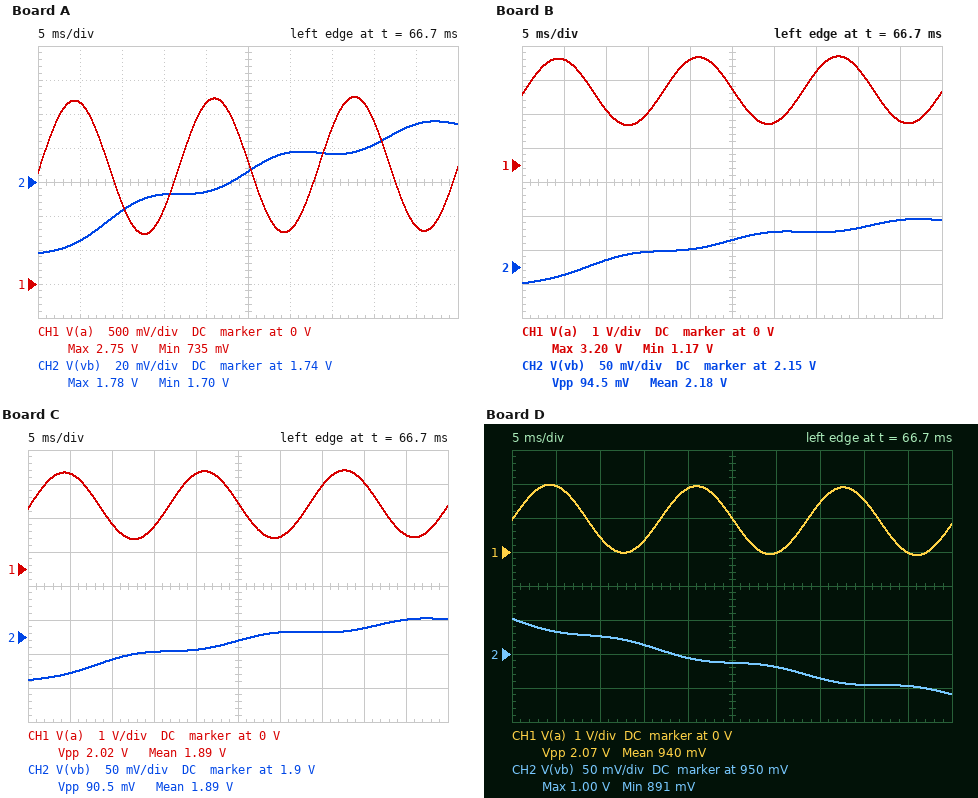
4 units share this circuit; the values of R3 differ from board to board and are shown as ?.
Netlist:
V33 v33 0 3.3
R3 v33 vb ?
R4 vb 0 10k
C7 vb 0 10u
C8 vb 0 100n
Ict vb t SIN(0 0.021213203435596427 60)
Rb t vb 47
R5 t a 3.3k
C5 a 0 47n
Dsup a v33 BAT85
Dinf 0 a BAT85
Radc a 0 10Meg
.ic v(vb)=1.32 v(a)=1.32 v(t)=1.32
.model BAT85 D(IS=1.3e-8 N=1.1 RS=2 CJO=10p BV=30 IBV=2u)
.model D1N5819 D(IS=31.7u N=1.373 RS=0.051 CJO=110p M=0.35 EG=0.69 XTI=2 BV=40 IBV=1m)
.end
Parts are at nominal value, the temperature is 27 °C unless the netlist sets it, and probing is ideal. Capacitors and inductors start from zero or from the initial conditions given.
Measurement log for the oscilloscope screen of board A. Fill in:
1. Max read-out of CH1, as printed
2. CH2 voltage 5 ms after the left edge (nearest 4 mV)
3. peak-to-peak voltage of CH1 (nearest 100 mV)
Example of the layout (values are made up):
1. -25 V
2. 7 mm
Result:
1. 2.75 V
2. 1.704 V
3. 2.0 V
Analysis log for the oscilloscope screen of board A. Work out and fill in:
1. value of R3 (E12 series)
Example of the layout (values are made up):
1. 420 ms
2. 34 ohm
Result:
1. 8.2 kΩ
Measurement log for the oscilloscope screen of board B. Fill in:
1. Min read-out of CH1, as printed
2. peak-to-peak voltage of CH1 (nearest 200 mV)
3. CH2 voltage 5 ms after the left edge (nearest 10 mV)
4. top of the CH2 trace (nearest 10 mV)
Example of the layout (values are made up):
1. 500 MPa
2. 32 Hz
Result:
1. 1.17 V
2. 2.0 V
3. 2.14 V
4. 2.22 V
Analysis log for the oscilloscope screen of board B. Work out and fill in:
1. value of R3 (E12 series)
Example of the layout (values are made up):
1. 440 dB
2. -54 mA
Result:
1. 4.7 kΩ
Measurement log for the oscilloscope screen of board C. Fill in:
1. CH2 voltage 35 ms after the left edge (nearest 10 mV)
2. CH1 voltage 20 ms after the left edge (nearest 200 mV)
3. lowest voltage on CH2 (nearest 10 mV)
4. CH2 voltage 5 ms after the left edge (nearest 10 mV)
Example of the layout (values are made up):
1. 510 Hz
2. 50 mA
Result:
1. 1.91 V
2. 2.8 V
3. 1.84 V
4. 1.85 V
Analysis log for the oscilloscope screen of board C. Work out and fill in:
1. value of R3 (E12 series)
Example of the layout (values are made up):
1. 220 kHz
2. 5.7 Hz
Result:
1. 6.8 kΩ
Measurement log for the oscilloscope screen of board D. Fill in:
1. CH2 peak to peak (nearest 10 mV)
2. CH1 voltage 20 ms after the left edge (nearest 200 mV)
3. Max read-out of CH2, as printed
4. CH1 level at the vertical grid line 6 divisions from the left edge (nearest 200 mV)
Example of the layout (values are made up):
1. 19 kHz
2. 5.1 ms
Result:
1. 110 mV
2. 1.8 V
3. 1.00 V
4. 0 V
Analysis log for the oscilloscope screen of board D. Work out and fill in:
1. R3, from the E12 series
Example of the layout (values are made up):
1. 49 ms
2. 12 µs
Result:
1. 33 kΩ
